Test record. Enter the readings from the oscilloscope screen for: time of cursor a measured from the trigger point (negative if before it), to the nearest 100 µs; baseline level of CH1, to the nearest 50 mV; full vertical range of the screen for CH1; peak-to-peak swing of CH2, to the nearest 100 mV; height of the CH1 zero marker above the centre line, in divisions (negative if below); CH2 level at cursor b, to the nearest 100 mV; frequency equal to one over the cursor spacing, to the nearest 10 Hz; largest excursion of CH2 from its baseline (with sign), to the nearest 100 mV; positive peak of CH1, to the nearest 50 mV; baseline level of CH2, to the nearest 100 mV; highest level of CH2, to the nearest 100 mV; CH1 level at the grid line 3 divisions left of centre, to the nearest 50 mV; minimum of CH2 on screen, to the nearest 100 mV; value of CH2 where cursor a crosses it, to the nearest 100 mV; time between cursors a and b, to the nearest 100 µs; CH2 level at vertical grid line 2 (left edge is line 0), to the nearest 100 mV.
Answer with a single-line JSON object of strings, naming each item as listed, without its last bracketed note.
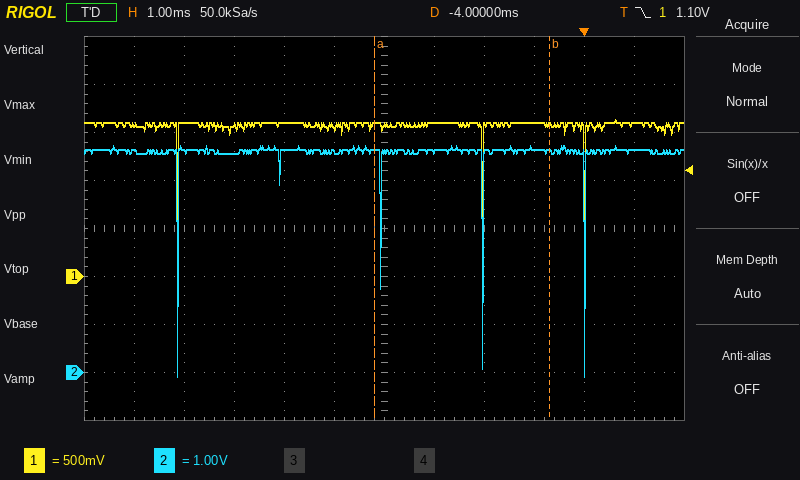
{"time of cursor a measured from the trigger point (negative if before it), to the nearest 100 µs": "-4.2 ms", "baseline level of CH1, to the nearest 50 mV": "1.60 V", "full vertical range of the screen for CH1": "4 V", "peak-to-peak swing of CH2, to the nearest 100 mV": "4.8 V", "height of the CH1 zero marker above the centre line, in divisions": "-1.0 div", "CH2 level at cursor b, to the nearest 100 mV": "4.6 V", "frequency equal to one over the cursor spacing, to the nearest 10 Hz": "290 Hz", "largest excursion of CH2 from its baseline (with sign), to the nearest 100 mV": "-4.7 V", "positive peak of CH1, to the nearest 50 mV": "1.65 V", "baseline level of CH2, to the nearest 100 mV": "4.6 V", "highest level of CH2, to the nearest 100 mV": "4.7 V", "CH1 level at the grid line 3 divisions left of centre, to the nearest 50 mV": "1.55 V", "minimum of CH2 on screen, to the nearest 100 mV": "-100 mV", "value of CH2 where cursor a crosses it, to the nearest 100 mV": "4.6 V", "time between cursors a and b, to the nearest 100 µs": "3.5 ms", "CH2 level at vertical grid line 2 (left edge is line 0), to the nearest 100 mV": "4.6 V"}
